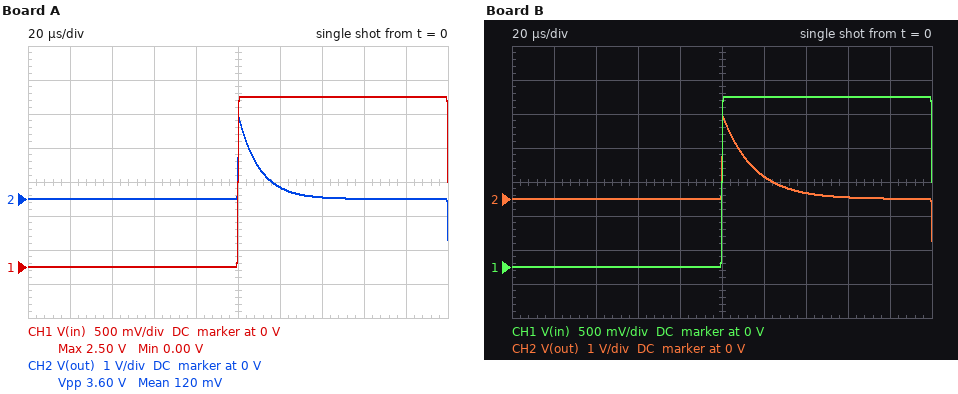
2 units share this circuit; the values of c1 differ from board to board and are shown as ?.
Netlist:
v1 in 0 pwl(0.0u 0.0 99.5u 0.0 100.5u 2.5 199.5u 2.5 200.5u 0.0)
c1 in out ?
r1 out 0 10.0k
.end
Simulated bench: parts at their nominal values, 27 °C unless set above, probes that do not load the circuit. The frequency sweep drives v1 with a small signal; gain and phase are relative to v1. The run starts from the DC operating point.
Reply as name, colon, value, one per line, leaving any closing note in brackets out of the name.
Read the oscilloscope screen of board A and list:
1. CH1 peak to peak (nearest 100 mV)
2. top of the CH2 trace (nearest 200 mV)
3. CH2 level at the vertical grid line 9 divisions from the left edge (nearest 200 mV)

CH1 peak to peak: 2.5 V
top of the CH2 trace: 2.4 V
CH2 level at the vertical grid line 9 divisions from the left edge: 0 V
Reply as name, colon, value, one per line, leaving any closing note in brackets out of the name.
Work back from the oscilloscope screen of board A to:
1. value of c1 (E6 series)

value of c1: 1 nF
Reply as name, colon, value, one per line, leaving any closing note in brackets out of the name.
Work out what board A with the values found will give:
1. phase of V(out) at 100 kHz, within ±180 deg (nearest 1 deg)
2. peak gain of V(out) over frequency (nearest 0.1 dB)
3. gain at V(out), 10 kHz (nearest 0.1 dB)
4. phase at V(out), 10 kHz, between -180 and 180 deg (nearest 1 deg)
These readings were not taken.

phase of V(out) at 100 kHz, within ±180 deg: 9 deg
peak gain of V(out) over frequency: 0 dB
gain at V(out), 10 kHz: -5.5 dB
phase at V(out), 10 kHz, between -180 and 180 deg: 58 deg
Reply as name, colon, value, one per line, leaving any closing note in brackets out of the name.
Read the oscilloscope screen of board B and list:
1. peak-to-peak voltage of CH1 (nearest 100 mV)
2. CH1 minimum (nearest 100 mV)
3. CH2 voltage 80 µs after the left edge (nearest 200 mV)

peak-to-peak voltage of CH1: 2.5 V
CH1 minimum: 0 V
CH2 voltage 80 µs after the left edge: 0 V
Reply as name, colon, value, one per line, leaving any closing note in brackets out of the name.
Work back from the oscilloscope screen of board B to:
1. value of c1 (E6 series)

value of c1: 1.5 nF
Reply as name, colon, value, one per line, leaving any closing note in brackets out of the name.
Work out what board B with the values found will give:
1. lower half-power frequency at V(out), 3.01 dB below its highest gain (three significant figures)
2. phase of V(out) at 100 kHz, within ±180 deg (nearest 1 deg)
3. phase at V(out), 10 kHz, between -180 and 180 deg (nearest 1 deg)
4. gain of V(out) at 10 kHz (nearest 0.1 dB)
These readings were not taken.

lower half-power frequency at V(out), 3.01 dB below its highest gain: 10.6 kHz
phase of V(out) at 100 kHz, within ±180 deg: 6 deg
phase at V(out), 10 kHz, between -180 and 180 deg: 47 deg
gain of V(out) at 10 kHz: -3.3 dB
